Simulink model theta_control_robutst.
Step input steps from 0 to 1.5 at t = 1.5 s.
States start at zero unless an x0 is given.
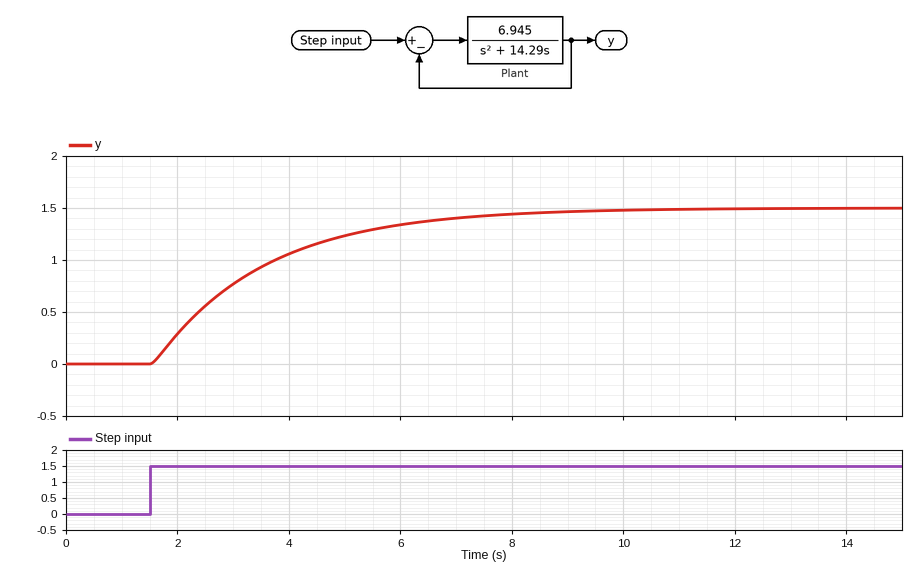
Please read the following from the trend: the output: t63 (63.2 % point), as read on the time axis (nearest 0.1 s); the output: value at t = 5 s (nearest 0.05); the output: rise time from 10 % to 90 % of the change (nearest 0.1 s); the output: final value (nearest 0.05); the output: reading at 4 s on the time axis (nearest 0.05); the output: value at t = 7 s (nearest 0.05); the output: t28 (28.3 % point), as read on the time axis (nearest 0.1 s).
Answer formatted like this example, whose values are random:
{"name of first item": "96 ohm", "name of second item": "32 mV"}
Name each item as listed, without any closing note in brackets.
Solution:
{"the output: t63 (63.2 % point), as read on the time axis": "3.6 s", "the output: value at t = 5 s": "1.25", "the output: rise time from 10 % to 90 % of the change": "4.4 s", "the output: final value": "1.50", "the output: reading at 4 s on the time axis": "1.05", "the output: value at t = 7 s": "1.40", "the output: t28 (28.3 % point), as read on the time axis": "2.2 s"}
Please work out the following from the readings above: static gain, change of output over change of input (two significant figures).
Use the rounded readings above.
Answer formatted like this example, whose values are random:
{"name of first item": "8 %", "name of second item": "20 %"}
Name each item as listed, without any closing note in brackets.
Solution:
{"static gain, change of output over change of input": "1.0"}
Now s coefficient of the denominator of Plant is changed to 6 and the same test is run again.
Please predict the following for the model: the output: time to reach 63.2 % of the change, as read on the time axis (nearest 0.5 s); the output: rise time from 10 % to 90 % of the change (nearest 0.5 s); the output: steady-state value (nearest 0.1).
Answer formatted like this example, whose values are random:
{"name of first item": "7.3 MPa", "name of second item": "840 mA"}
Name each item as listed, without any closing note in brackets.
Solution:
{"the output: time to reach 63.2 % of the change, as read on the time axis": "2.5 s", "the output: rise time from 10 % to 90 % of the change": "1.5 s", "the output: steady-state value": "1.5"}
